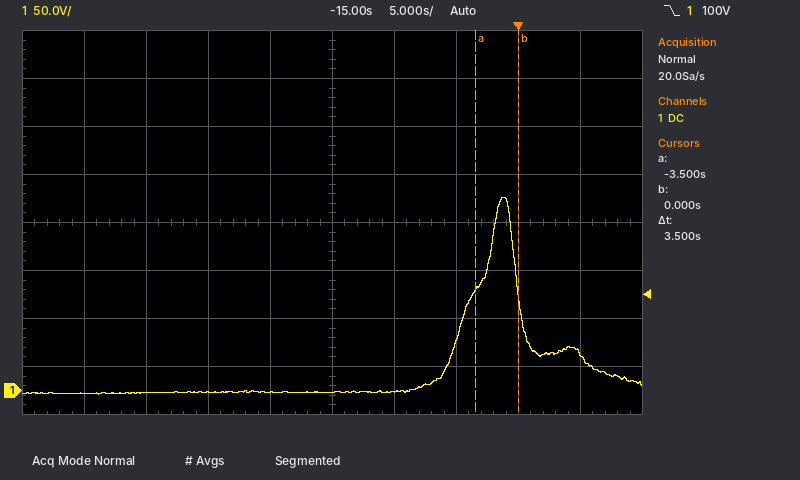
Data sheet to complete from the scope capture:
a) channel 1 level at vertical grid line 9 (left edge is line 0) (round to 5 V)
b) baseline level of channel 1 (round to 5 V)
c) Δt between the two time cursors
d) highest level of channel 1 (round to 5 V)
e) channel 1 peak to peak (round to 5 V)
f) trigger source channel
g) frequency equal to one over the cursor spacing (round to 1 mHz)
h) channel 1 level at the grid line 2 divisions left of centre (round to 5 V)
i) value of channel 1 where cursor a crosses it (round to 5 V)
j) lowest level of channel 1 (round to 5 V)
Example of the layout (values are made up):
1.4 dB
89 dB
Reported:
40 V
0 V
3.5 s
200 V
205 V
channel 1
286 mHz
0 V
105 V
-5 V
